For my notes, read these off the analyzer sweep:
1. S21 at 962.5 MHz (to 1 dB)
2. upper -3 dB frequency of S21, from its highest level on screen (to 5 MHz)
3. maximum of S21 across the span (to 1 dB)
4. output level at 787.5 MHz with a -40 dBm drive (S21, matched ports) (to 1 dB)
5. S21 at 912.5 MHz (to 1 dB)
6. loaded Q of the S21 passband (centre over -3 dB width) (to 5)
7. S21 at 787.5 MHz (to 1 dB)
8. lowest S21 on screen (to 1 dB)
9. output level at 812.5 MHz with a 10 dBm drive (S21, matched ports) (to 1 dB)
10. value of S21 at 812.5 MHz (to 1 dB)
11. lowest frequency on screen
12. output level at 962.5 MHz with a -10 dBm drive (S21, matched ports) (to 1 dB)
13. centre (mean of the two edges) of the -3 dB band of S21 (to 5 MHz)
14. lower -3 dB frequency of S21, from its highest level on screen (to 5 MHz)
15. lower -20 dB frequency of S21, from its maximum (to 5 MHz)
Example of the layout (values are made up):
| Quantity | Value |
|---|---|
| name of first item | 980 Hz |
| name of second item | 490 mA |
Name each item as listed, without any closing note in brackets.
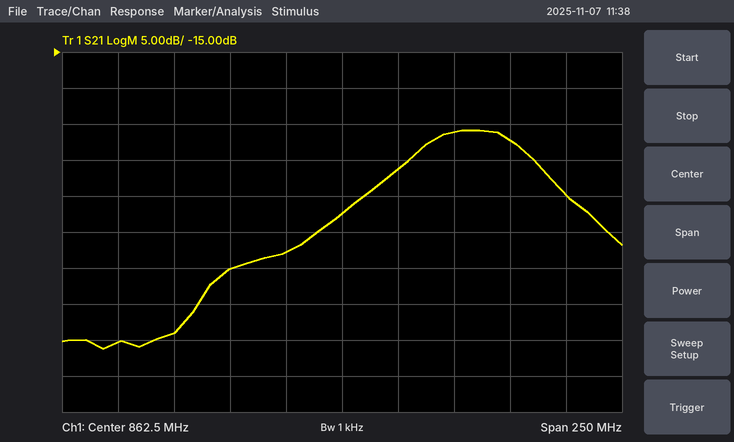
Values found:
| Quantity | Value |
|---|---|
| S21 at 962.5 MHz | -35 dB |
| upper -3 dB frequency of S21, from its highest level on screen | 945 MHz |
| maximum of S21 across the span | -26 dB |
| output level at 787.5 MHz with a -40 dBm drive (S21, matched ports) | -94 dBm |
| S21 at 912.5 MHz | -26 dB |
| loaded Q of the S21 passband (centre over -3 dB width) | 20 |
| S21 at 787.5 MHz | -54 dB |
| lowest S21 on screen | -56 dB |
| output level at 812.5 MHz with a 10 dBm drive (S21, matched ports) | -35 dBm |
| value of S21 at 812.5 MHz | -45 dB |
| lowest frequency on screen | 737.5 MHz |
| output level at 962.5 MHz with a -10 dBm drive (S21, matched ports) | -45 dBm |
| centre (mean of the two edges) of the -3 dB band of S21 | 920 MHz |
| lower -3 dB frequency of S21, from its highest level on screen | 895 MHz |
| lower -20 dB frequency of S21, from its maximum | 810 MHz |
